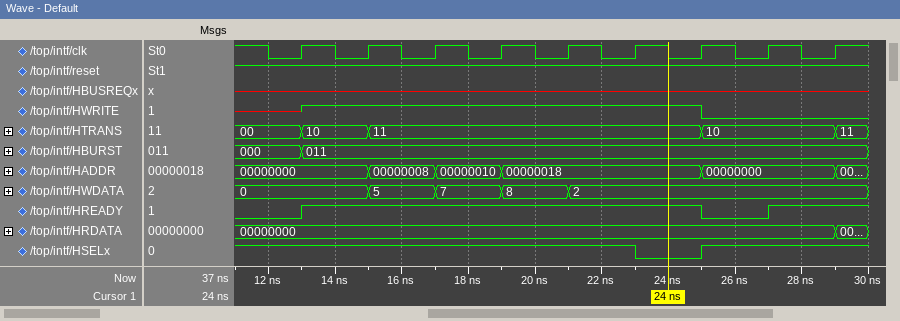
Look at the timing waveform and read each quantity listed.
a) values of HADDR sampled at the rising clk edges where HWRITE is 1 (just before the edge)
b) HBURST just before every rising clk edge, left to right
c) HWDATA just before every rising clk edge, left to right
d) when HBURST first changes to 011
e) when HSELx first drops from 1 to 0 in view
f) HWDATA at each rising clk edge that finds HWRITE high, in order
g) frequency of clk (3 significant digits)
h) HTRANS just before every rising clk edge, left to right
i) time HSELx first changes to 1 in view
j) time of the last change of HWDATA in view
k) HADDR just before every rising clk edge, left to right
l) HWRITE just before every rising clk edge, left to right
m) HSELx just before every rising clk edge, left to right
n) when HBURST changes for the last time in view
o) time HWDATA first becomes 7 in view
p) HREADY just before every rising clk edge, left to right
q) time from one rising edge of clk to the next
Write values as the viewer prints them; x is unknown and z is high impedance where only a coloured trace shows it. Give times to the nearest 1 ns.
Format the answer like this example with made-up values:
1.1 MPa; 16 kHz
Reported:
00000000, 00000008, 00000010, 00000018, 00000018, 00000018; 000, 011, 011, 011, 011, 011, 011, 011, 011; 0, 0, 5, 7, 8, 2, 2, 2, 2; 13 ns; 23 ns; 0, 5, 7, 8, 2, 2; 500 MHz; 00, 10, 11, 11, 11, 11, 11, 10, 10; 25 ns; 21 ns; 00000000, 00000000, 00000008, 00000010, 00000018, 00000018, 00000018, 00000000, 00000000; x 1 1 1 1 1 1 0 0; 1 1 1 1 1 1 0 1 1; 13 ns; 17 ns; 0 1 1 1 1 1 1 0 1; 2 ns
